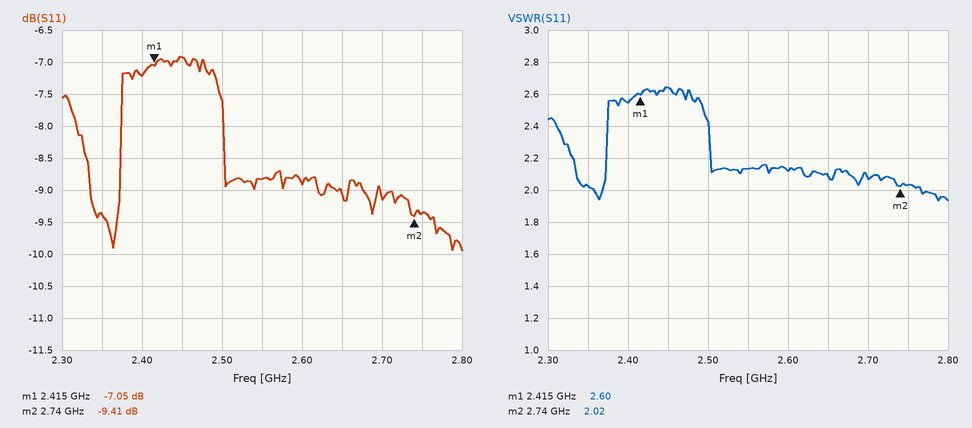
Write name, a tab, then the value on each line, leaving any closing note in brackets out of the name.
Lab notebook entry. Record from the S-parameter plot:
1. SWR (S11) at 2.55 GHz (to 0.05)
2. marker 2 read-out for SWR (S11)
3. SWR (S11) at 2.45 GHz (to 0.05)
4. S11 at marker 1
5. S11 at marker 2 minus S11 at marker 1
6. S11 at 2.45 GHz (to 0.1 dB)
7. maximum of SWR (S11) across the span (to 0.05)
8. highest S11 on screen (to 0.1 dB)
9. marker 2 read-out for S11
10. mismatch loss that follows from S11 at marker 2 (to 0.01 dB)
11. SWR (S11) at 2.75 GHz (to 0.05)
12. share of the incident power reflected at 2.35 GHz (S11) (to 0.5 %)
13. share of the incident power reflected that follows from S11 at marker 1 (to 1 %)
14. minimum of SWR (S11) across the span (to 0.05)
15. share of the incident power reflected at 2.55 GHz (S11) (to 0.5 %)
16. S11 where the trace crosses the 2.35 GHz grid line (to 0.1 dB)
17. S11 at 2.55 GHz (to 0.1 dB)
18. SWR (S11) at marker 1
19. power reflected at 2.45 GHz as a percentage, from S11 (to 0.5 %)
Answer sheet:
SWR (S11) at 2.55 GHz	2.15
marker 2 read-out for SWR	2.02
SWR (S11) at 2.45 GHz	2.65
S11 at marker 1	-7.05 dB
S11 at marker 2 minus S11 at marker 1	-2.36 dB
S11 at 2.45 GHz	-6.9 dB
maximum of SWR (S11) across the span	2.65
highest S11 on screen	-6.9 dB
marker 2 read-out for S11	-9.41 dB
mismatch loss that follows from S11 at marker 2	0.53 dB
SWR (S11) at 2.75 GHz	2.05
share of the incident power reflected at 2.35 GHz (S11)	11.5 %
share of the incident power reflected that follows from S11 at marker 1	20 %
minimum of SWR (S11) across the span	1.95
share of the incident power reflected at 2.55 GHz (S11)	13.0 %
S11 where the trace crosses the 2.35 GHz grid line	-9.4 dB
S11 at 2.55 GHz	-8.8 dB
SWR (S11) at marker 1	2.60
power reflected at 2.45 GHz as a percentage, from S11	20.5 %
